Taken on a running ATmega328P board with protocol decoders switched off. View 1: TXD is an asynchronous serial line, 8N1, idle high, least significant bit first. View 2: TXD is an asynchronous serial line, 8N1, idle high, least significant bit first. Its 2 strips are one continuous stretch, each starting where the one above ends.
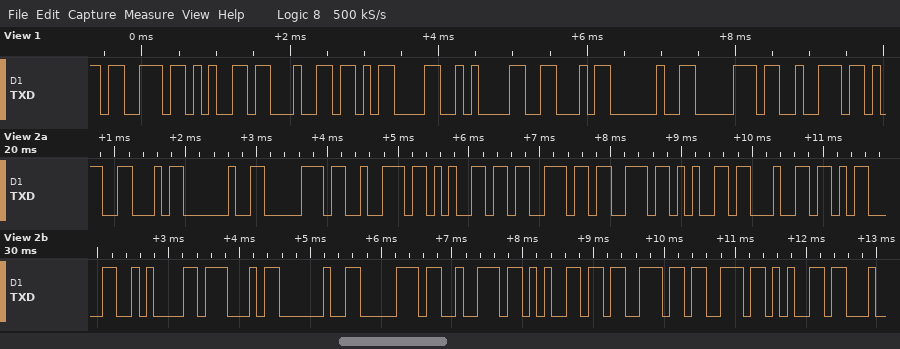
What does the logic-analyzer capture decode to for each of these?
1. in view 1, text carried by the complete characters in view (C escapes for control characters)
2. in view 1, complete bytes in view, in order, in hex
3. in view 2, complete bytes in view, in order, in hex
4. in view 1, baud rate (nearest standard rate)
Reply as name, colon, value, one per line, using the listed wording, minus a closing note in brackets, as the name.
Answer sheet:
in view 1, text carried by the complete characters in view: "sed\r\nF pr"
in view 1, complete bytes in view, in order, in hex: 73 65 64 0D 0A 46 20 70 72
in view 2, complete bytes in view, in order, in hex: 0x46 0x20 0x70 0x72 0x65 0x73 0x73 0x65 0x64 0x0D 0x0A 0x47 0x20 0x70 0x72 0x65 0x73 0x73 0x65
in view 1, baud rate: 9600 baud
